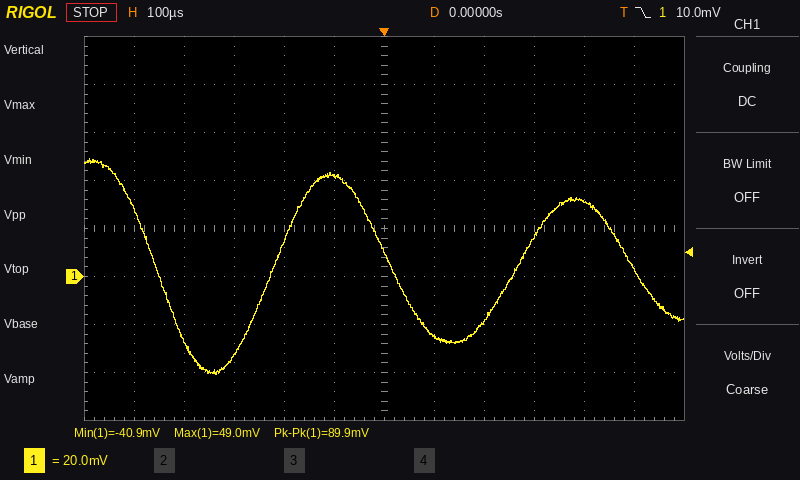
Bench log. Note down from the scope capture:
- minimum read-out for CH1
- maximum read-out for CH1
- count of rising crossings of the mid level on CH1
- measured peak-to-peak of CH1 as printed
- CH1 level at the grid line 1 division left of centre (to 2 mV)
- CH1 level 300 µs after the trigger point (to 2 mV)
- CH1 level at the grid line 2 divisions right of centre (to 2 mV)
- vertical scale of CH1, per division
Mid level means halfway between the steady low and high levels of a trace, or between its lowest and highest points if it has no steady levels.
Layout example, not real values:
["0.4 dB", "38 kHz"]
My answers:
["-40.9 mV", "49.0 mV", "2", "89.9 mV", "42 mV", "16 mV", "-18 mV", "20 mV"]
